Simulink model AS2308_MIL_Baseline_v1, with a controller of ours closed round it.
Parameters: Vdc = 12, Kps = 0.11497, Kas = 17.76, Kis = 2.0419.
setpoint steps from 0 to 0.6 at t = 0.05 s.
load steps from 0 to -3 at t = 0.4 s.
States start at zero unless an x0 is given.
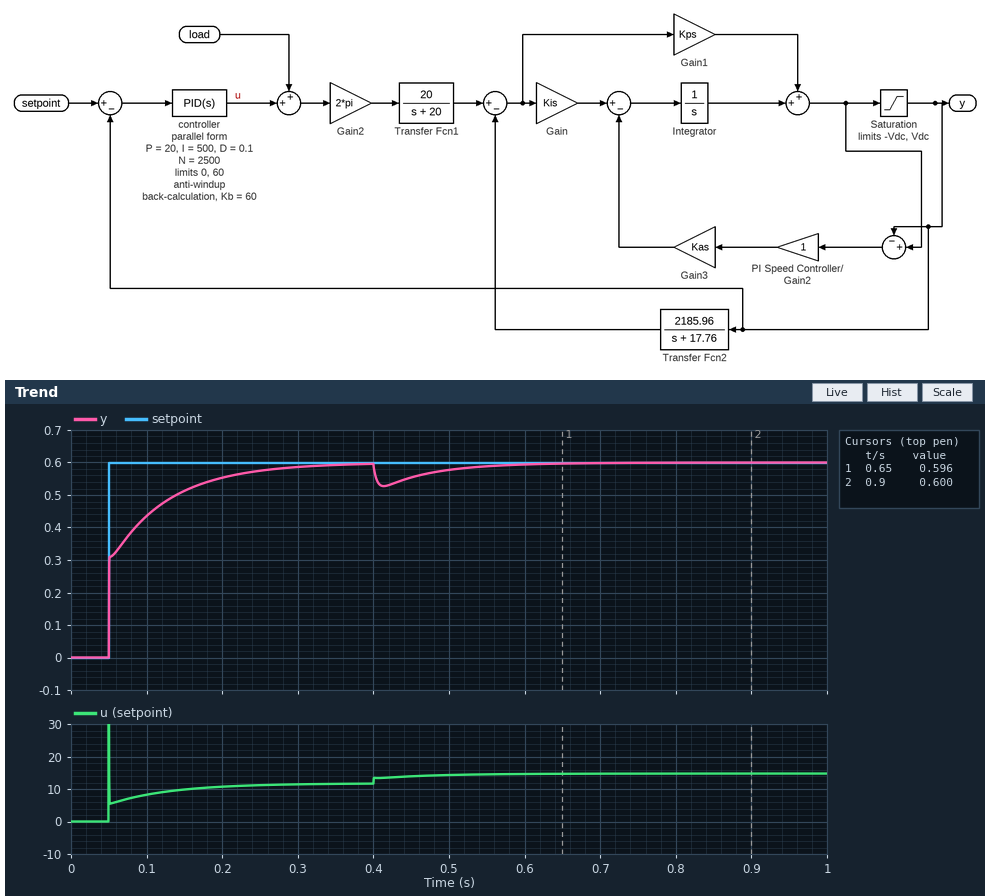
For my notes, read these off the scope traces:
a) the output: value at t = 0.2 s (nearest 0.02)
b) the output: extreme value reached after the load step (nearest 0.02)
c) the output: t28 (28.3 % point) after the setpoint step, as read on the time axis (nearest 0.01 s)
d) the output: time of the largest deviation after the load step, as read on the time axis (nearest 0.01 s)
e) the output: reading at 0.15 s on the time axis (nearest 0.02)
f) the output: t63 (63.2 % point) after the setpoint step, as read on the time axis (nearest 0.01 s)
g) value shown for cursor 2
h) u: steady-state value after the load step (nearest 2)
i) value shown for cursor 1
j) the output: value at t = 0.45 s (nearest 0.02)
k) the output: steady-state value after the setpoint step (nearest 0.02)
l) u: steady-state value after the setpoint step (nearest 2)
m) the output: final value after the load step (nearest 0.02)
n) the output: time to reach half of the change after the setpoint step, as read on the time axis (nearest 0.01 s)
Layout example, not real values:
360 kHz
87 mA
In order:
0.56
0.52
0.05 s
0.41 s
0.52
0.08 s
0.600
14
0.596
0.56
0.60
12
0.60
0.05 s
